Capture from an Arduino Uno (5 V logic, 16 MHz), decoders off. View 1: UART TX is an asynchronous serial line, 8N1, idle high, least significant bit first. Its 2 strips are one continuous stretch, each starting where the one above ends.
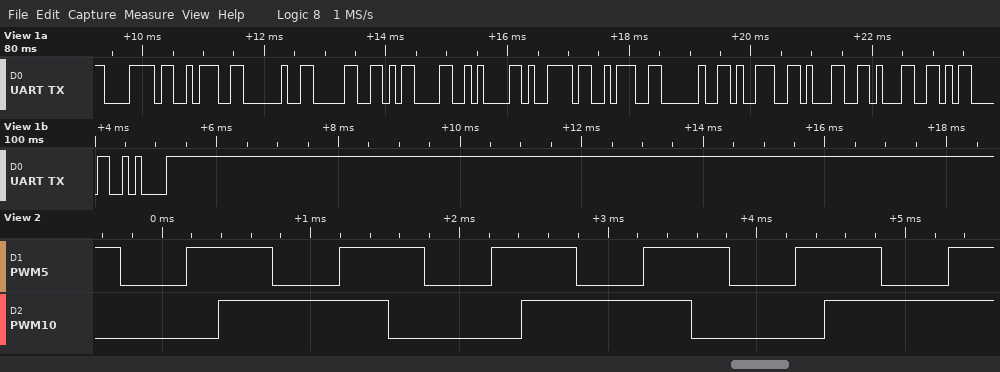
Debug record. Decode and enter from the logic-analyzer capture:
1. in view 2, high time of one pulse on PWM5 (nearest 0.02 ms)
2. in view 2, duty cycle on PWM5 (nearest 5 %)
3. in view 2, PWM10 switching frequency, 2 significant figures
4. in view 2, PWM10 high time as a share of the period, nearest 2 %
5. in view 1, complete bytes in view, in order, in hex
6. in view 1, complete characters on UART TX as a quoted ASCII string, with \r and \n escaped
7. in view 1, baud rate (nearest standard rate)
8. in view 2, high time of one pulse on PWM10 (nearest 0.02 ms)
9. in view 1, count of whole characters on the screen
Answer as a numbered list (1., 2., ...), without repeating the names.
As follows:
1. 0.58 ms
2. 55 %
3. 490 Hz
4. 56 %
5. 78 3A 20 30 0D 0A 79 3A 20 39 31 31 0D 0A
6. "x: 0\r\ny: 911\r\n"
7. 9600 baud
8. 1.14 ms
9. 14
